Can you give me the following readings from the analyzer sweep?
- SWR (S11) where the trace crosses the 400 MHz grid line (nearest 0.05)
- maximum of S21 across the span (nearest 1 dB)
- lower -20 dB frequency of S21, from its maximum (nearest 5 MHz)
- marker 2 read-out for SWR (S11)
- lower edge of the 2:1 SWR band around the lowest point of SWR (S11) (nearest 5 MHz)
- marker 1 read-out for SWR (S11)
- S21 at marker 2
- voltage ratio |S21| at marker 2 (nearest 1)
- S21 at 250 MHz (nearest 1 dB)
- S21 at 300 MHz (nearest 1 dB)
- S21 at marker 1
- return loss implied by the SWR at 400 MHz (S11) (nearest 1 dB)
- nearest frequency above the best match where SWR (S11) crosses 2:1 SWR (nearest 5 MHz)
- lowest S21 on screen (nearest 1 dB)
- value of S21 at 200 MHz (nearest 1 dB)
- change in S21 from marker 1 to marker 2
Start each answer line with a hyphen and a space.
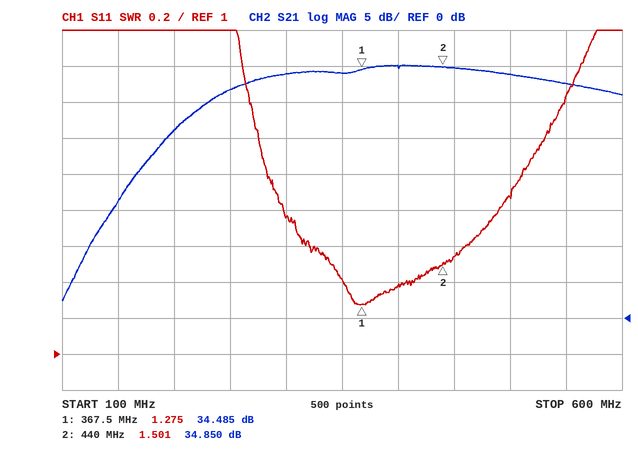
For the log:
- 1.40
- 35 dB
- 145 MHz
- 1.501
- 285 MHz
- 1.275
- 34.850 dB
- 55
- 32 dB
- 34 dB
- 34.485 dB
- 16 dB
- 510 MHz
- 2 dB
- 26 dB
- 0.365 dB
